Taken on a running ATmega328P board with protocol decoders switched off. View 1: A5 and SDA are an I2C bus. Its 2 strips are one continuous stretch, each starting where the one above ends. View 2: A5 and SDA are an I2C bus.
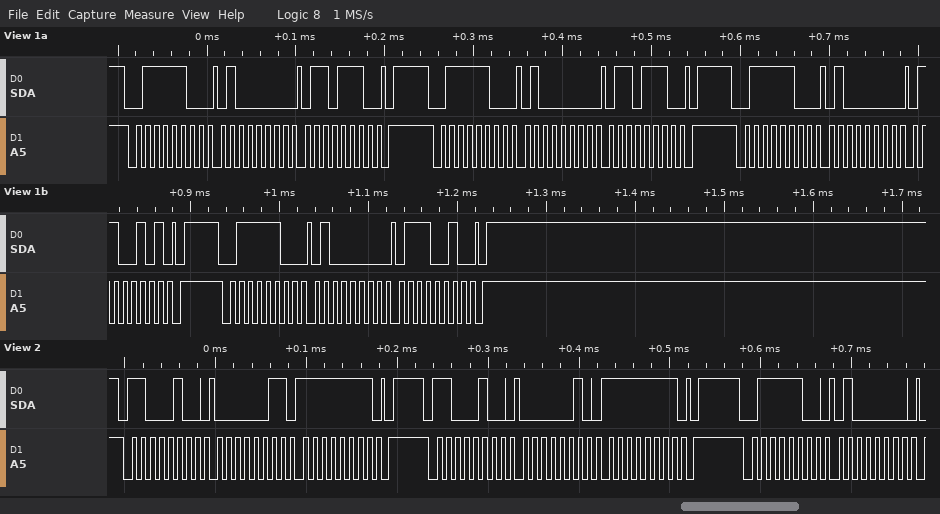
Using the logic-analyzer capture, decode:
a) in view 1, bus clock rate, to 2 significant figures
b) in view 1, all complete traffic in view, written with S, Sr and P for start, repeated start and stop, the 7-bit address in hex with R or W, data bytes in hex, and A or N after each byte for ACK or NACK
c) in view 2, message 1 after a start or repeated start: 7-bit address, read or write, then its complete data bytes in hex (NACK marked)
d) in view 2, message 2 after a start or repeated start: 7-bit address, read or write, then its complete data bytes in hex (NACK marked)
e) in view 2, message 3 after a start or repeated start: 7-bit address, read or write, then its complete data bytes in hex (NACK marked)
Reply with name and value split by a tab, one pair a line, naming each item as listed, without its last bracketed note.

in view 1, bus clock rate, to 2 significant figures	100 kHz
in view 1, all complete traffic in view, written with S, Sr and P for start, repeated start and stop, the 7-bit address in hex with R or W, data bytes in hex, and A or N after each byte for ACK or NACK	S 3EW A 40 A 6E A P S 3EW A 40 A 6E A P S 3EW A 40 A 65 A P S 3EW A 40 A 72 A P
in view 2, message 1 after a start or repeated start: 7-bit address, read or write, then its complete data bytes in hex	0x62 write: 03 FF
in view 2, message 2 after a start or repeated start: 7-bit address, read or write, then its complete data bytes in hex	0x62 write: 02 FF
in view 2, message 3 after a start or repeated start: 7-bit address, read or write, then its complete data bytes in hex	0x3E write: 40
